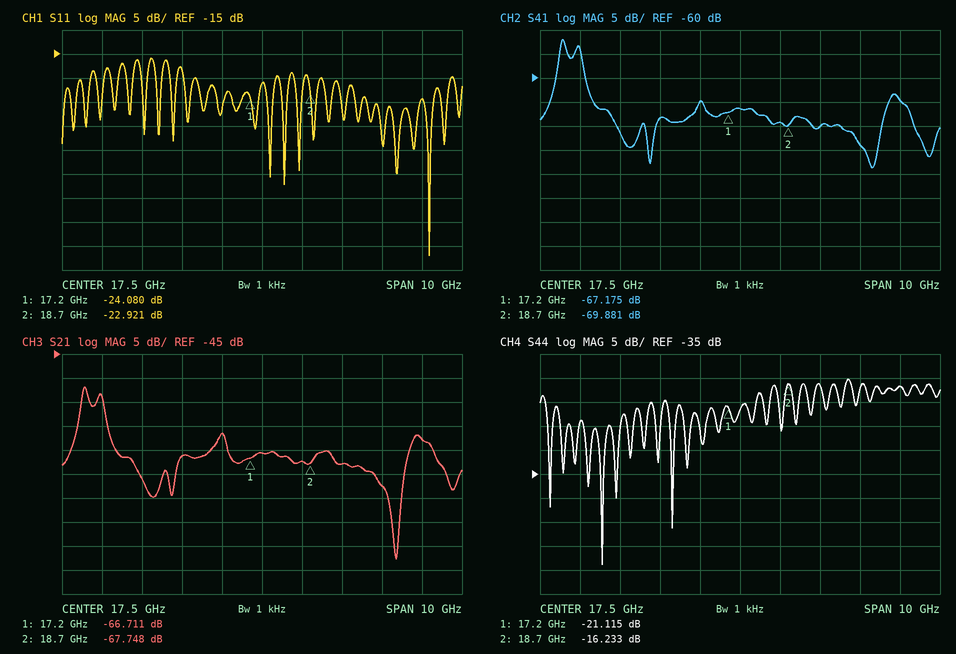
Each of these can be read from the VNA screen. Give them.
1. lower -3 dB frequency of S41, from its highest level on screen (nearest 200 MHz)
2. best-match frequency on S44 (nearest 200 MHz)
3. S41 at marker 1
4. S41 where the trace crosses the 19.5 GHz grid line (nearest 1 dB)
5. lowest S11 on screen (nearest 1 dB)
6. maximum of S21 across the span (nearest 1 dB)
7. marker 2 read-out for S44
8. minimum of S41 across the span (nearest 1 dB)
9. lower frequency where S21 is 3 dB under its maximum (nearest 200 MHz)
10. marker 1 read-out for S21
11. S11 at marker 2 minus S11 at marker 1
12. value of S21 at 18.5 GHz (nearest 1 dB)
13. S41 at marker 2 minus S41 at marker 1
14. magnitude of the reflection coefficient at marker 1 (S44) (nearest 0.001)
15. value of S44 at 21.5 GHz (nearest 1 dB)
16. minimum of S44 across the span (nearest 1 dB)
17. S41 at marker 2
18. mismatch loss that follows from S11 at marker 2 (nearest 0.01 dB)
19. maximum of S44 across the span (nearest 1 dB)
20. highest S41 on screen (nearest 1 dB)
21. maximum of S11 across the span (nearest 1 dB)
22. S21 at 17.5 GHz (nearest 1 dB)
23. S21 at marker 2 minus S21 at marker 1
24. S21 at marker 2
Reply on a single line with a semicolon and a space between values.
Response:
13.0 GHz; 14.0 GHz; -67.175 dB; -70 dB; -57 dB; -52 dB; -16.233 dB; -79 dB; 13.0 GHz; -66.711 dB; 1.159 dB; -67 dB; -2.706 dB; 0.088; -17 dB; -54 dB; -69.881 dB; 0.02 dB; -15 dB; -52 dB; -16 dB; -66 dB; -1.037 dB; -67.748 dB
